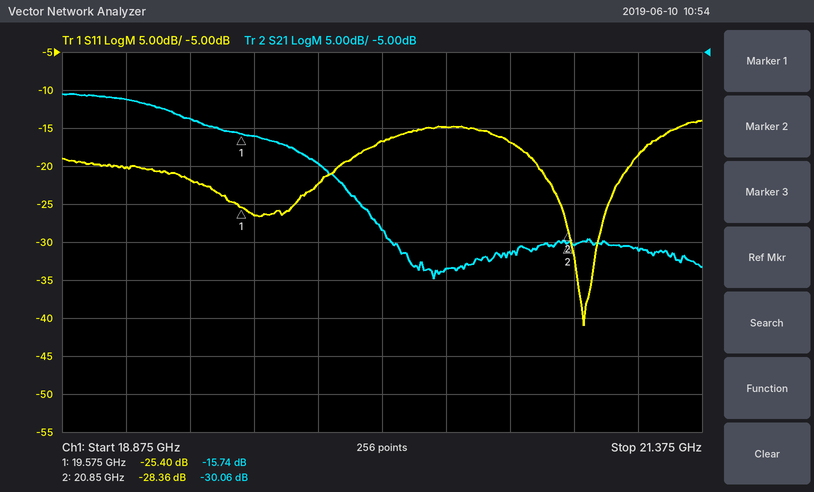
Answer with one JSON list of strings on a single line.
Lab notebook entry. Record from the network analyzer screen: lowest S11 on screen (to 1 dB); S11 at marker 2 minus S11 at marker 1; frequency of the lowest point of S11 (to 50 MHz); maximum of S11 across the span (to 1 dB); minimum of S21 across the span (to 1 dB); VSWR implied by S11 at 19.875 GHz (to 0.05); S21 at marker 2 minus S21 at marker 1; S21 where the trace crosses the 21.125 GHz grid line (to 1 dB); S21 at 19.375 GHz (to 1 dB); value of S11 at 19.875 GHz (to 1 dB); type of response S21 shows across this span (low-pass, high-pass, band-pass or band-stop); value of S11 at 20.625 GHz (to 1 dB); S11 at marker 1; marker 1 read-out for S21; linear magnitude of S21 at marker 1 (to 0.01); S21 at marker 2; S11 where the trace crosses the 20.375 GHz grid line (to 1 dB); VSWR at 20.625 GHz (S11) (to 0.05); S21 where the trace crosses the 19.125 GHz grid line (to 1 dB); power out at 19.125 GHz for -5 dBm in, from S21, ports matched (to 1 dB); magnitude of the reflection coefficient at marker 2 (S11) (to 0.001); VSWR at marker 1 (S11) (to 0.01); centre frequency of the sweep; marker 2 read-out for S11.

["-41 dB", "-2.96 dB", "20.90 GHz", "-14 dB", "-35 dB", "1.15", "-14.32 dB", "-31 dB", "-14 dB", "-22 dB", "low-pass", "-17 dB", "-25.40 dB", "-15.74 dB", "0.16", "-30.06 dB", "-15 dB", "1.35", "-11 dB", "-16 dBm", "0.038", "1.11", "20.125 GHz", "-28.36 dB"]
